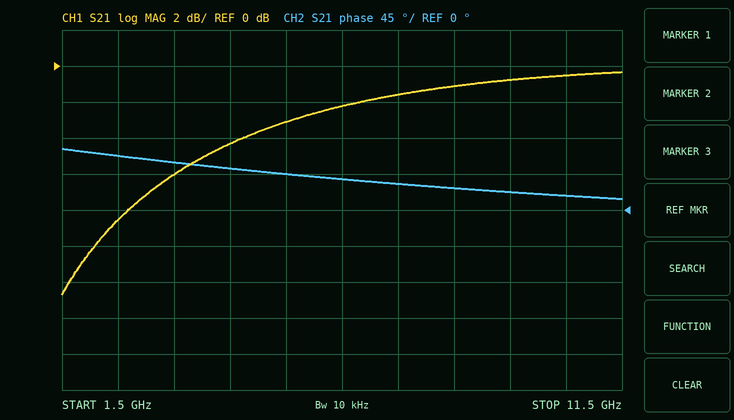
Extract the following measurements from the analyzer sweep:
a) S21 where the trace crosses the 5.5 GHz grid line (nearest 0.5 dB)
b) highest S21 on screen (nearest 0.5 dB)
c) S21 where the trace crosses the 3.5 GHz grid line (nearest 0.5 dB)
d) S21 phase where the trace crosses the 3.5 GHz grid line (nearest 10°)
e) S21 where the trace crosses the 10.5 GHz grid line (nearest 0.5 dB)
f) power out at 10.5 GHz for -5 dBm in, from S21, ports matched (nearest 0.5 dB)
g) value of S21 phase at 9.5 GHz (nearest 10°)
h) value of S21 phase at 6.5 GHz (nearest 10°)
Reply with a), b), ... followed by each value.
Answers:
a) -3.0 dB
b) -0.5 dB
c) -6.0 dB
d) 60°
e) -0.5 dB
f) -5.5 dBm
g) 20°
h) 40°
